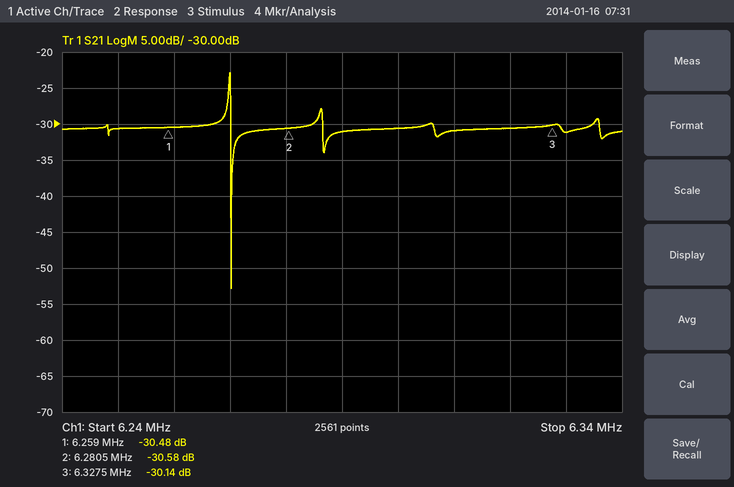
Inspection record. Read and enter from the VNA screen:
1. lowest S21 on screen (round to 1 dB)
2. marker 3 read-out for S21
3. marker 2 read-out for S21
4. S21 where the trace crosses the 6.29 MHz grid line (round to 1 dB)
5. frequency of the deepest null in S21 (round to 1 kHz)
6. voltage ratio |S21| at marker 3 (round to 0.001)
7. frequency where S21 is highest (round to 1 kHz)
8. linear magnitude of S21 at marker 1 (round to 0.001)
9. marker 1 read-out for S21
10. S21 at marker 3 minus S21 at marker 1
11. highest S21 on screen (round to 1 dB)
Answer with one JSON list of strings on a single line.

["-53 dB", "-30.14 dB", "-30.58 dB", "-31 dB", "6.270 MHz", "0.031", "6.270 MHz", "0.030", "-30.48 dB", "0.34 dB", "-23 dB"]
